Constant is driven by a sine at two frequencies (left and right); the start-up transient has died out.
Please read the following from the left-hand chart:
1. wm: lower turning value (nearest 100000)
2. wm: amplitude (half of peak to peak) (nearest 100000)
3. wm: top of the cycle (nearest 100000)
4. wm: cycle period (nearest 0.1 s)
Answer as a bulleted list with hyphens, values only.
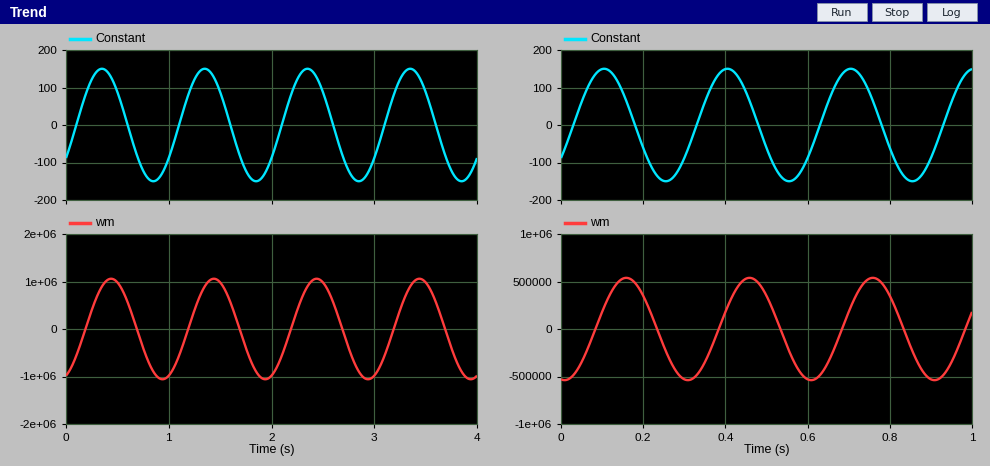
- -1100000
- 1100000
- 1100000
- 1.0 s
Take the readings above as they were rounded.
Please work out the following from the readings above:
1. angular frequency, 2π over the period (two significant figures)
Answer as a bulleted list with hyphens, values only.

- 6.3 rad/s
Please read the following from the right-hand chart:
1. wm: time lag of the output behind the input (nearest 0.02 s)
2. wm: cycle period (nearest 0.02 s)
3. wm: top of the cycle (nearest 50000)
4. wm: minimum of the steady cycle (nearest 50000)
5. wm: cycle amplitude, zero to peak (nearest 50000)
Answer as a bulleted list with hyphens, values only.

- 0.06 s
- 0.30 s
- 550000
- -550000
- 550000
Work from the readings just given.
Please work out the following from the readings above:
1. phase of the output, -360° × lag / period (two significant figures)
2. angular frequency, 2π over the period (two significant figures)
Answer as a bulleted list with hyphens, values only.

- -72°
- 21 rad/s
